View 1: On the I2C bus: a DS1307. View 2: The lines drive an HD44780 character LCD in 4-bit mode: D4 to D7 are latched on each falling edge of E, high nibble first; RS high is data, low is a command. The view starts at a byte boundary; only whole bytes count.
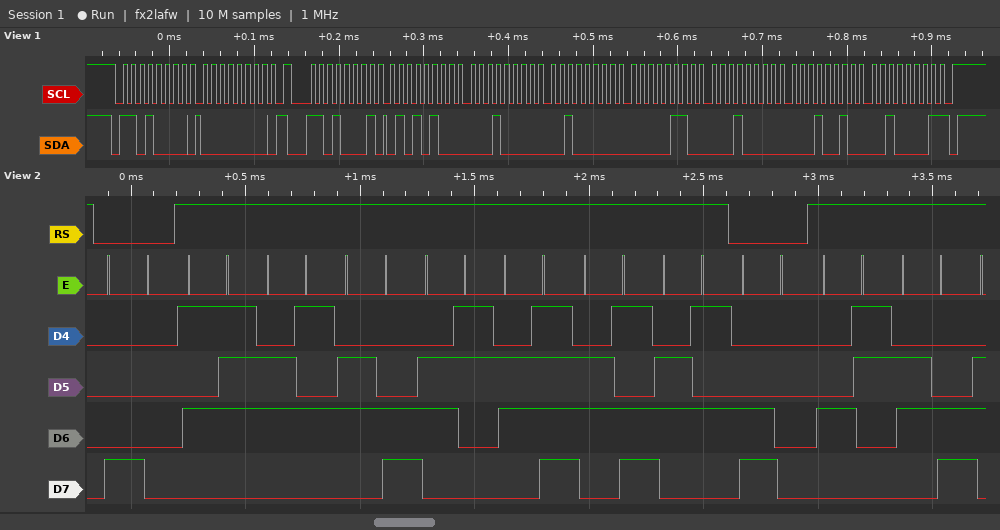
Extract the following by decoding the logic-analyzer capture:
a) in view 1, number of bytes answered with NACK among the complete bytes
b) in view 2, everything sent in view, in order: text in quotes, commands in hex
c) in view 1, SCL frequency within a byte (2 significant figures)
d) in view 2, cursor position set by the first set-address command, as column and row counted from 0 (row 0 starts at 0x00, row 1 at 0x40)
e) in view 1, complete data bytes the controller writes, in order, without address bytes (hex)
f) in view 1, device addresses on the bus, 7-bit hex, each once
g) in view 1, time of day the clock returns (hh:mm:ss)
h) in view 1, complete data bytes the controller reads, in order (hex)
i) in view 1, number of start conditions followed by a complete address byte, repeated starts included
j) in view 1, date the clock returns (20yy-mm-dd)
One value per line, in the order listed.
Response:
1
0x80 "Welcome" 0xC0 "Cl"
100 kHz
column 0, row 0
00
0x68
20:10:54
54 10 20 06 10 12 21
2
2021-12-10
